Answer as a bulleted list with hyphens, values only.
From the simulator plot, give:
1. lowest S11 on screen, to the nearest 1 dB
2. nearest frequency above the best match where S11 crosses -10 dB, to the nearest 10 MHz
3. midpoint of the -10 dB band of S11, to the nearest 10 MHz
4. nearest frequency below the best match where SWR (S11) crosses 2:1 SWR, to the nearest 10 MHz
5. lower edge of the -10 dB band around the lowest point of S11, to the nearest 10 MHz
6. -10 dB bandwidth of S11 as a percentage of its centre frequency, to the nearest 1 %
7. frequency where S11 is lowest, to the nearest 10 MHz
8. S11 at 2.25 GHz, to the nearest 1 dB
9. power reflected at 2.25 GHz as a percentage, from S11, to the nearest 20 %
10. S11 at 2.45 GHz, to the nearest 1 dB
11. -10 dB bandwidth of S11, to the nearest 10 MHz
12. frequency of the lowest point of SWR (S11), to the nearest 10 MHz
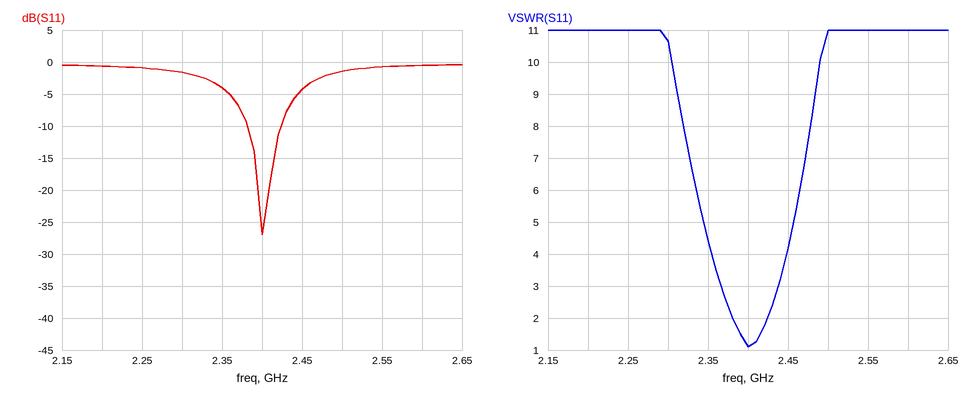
- -27 dB
- 2.42 GHz
- 2.40 GHz
- 2.38 GHz
- 2.38 GHz
- 2 %
- 2.40 GHz
- -1 dB
- 80 %
- -4 dB
- 40 MHz
- 2.40 GHz
